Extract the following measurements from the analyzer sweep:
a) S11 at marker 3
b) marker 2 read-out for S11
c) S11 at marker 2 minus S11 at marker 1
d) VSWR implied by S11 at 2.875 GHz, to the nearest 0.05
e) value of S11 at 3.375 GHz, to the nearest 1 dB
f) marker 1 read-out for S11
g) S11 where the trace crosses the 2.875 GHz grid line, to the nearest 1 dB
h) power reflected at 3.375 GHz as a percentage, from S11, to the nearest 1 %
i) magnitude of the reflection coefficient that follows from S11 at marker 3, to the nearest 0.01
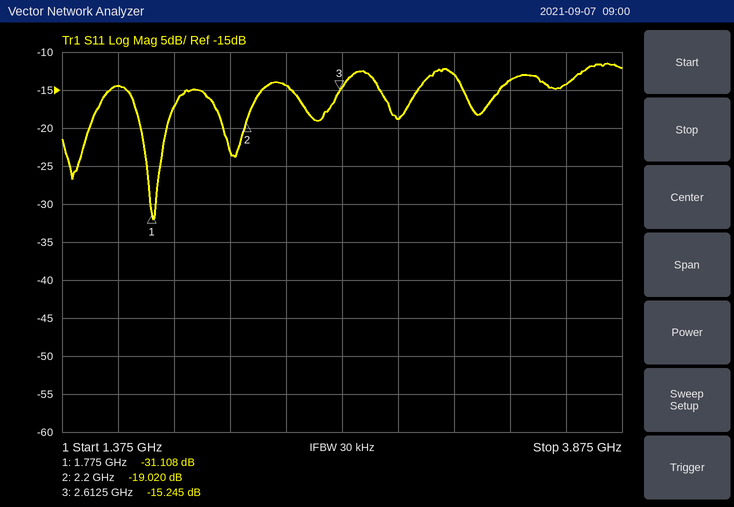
-15.245 dB
-19.020 dB
12.088 dB
1.25
-14 dB
-31.108 dB
-19 dB
4 %
0.17
